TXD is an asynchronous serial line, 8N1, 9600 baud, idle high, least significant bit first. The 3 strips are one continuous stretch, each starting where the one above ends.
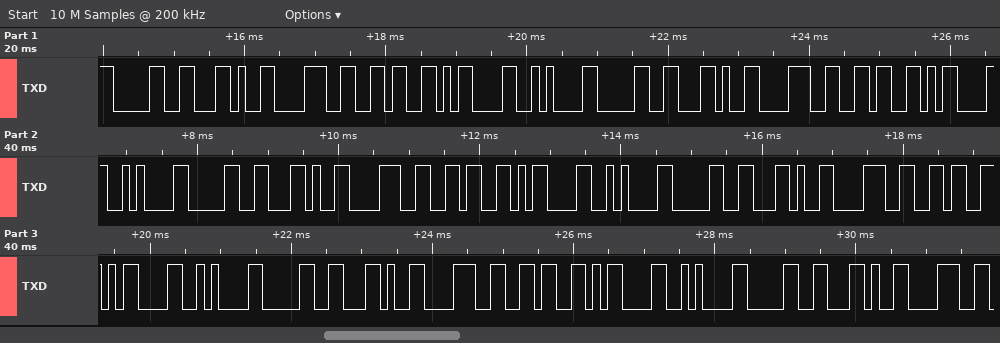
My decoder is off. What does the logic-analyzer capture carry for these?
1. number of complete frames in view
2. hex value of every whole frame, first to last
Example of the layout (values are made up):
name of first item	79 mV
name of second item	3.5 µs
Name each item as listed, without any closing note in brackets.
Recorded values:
number of complete frames in view	33
hex value of every whole frame, first to last	30 2C 38 36 0D 0A 30 2C 38 36 0D 0A 30 2C 38 36 0D 0A 30 2C 38 36 0D 0A 30 2C 38 36 0D 0A 30 2C 38
